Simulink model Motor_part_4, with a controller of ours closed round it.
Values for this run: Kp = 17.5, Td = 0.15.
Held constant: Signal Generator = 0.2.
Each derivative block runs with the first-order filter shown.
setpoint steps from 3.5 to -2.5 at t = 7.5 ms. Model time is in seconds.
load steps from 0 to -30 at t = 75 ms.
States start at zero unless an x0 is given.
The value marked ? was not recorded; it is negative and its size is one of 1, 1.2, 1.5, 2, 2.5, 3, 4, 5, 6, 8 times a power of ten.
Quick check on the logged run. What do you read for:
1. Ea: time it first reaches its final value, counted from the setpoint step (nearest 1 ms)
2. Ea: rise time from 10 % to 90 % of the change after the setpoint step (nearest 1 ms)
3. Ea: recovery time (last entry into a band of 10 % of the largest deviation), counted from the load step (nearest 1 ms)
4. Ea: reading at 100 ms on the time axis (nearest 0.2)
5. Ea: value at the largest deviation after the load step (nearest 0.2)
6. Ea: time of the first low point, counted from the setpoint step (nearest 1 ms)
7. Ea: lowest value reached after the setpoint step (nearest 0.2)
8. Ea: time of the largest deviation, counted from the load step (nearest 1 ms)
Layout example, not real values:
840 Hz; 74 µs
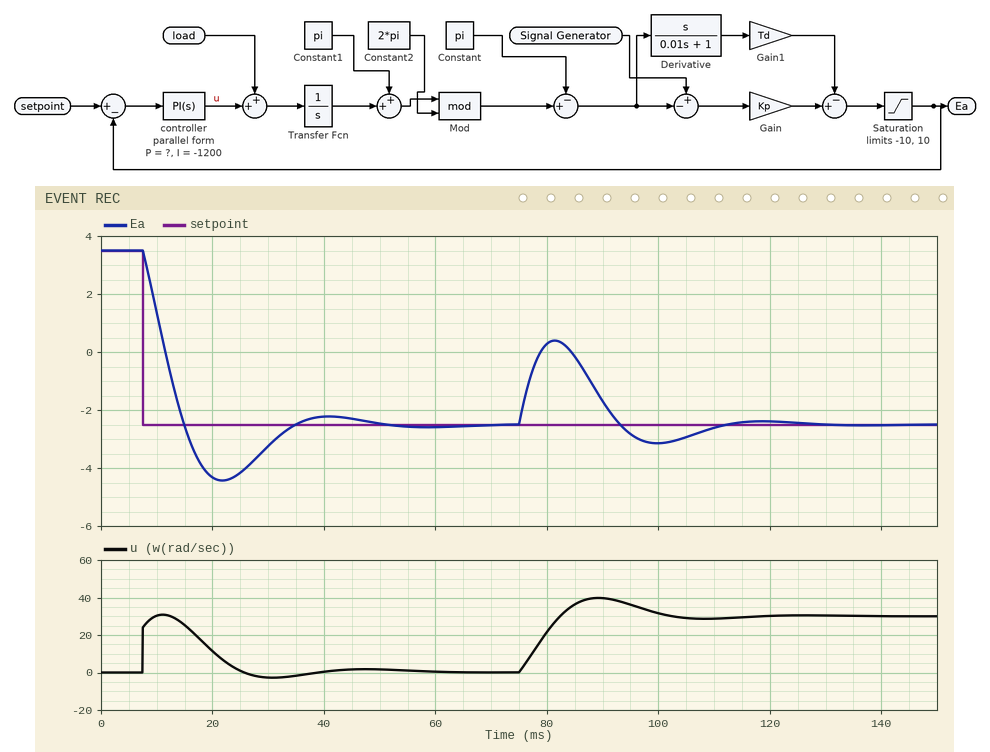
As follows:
7 ms; 6 ms; 32 ms; -3.2; 0.4; 14 ms; -4.4; 6 ms
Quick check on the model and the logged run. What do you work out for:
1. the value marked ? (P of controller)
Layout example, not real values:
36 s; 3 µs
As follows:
-4
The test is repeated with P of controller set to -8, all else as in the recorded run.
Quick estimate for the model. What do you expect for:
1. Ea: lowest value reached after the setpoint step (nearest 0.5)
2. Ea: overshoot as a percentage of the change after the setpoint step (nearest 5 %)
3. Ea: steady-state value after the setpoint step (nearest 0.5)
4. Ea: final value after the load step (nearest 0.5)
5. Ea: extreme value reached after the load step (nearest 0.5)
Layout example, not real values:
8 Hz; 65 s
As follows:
-3.5; 15 %; -2.5; -2.5; -0.5
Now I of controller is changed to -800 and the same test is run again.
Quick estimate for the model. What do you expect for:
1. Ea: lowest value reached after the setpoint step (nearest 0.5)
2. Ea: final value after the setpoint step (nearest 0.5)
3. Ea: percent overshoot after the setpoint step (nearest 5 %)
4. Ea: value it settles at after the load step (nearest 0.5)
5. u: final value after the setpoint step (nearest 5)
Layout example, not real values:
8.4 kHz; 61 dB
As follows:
-4.0; -2.5; 25 %; -2.5; 0
